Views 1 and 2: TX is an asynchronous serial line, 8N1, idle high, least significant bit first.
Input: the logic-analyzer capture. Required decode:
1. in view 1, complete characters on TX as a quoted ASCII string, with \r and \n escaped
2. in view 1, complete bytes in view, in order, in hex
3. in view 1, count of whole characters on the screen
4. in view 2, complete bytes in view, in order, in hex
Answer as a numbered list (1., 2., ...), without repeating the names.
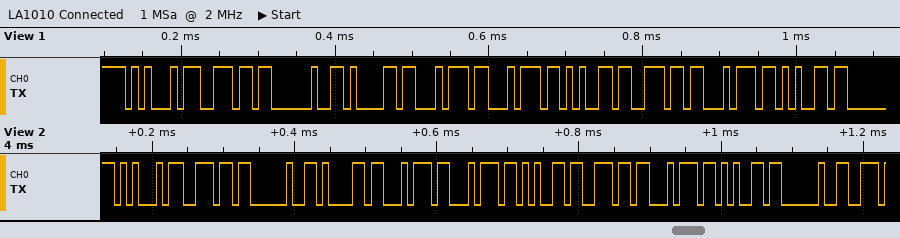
1. "En attente"
2. 45 6E 20 61 74 74 65 6E 74 65
3. 10
4. 45 6E 20 61 74 74 65 6E 74 65 20
